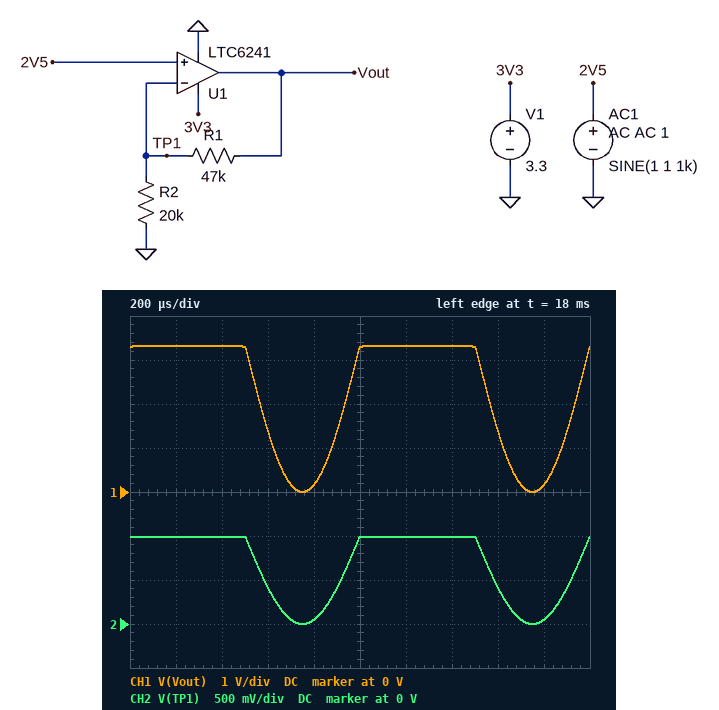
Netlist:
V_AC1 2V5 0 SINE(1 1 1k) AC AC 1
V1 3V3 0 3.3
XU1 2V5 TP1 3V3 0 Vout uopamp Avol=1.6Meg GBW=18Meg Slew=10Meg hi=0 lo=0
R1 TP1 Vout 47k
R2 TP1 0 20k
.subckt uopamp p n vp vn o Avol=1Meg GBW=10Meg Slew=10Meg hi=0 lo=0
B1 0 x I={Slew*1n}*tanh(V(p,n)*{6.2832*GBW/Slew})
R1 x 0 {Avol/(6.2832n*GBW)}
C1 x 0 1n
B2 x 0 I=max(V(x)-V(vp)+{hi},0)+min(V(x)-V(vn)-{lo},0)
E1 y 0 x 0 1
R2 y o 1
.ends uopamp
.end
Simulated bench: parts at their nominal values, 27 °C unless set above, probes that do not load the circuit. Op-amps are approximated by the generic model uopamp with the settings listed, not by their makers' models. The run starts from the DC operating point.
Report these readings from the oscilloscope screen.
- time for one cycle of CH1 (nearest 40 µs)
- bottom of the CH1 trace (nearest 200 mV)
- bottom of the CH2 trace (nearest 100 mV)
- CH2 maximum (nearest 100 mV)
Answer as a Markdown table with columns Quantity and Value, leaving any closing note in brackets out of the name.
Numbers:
| Quantity | Value |
|---|---|
| time for one cycle of CH1 | 1.00 ms |
| bottom of the CH1 trace | 0 V |
| bottom of the CH2 trace | 0 V |
| CH2 maximum | 1.0 V |
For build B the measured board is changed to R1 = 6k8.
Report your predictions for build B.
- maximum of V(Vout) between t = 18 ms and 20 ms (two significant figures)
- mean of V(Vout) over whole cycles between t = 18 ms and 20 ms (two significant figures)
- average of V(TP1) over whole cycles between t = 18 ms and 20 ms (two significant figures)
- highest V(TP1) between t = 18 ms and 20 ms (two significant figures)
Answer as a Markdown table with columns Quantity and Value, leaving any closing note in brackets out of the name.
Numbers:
| Quantity | Value |
|---|---|
| maximum of V(Vout) between t = 18 ms and 20 ms | 2.7 V |
| mean of V(Vout) over whole cycles between t = 18 ms and 20 ms | 1.3 V |
| average of V(TP1) over whole cycles between t = 18 ms and 20 ms | 1.0 V |
| highest V(TP1) between t = 18 ms and 20 ms | 2.0 V |
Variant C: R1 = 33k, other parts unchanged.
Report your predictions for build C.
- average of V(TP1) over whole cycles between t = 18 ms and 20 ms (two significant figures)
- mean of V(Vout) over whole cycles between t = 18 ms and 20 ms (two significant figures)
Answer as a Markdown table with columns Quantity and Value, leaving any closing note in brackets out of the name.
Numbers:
| Quantity | Value |
|---|---|
| average of V(TP1) over whole cycles between t = 18 ms and 20 ms | 800 mV |
| mean of V(Vout) over whole cycles between t = 18 ms and 20 ms | 2.1 V |
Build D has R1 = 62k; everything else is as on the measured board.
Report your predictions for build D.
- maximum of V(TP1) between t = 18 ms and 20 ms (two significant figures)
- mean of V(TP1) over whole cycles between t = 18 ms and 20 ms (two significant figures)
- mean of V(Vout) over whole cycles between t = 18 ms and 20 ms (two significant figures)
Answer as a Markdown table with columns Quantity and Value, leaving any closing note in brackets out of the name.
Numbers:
| Quantity | Value |
|---|---|
| maximum of V(TP1) between t = 18 ms and 20 ms | 810 mV |
| mean of V(TP1) over whole cycles between t = 18 ms and 20 ms | 580 mV |
| mean of V(Vout) over whole cycles between t = 18 ms and 20 ms | 2.4 V |
